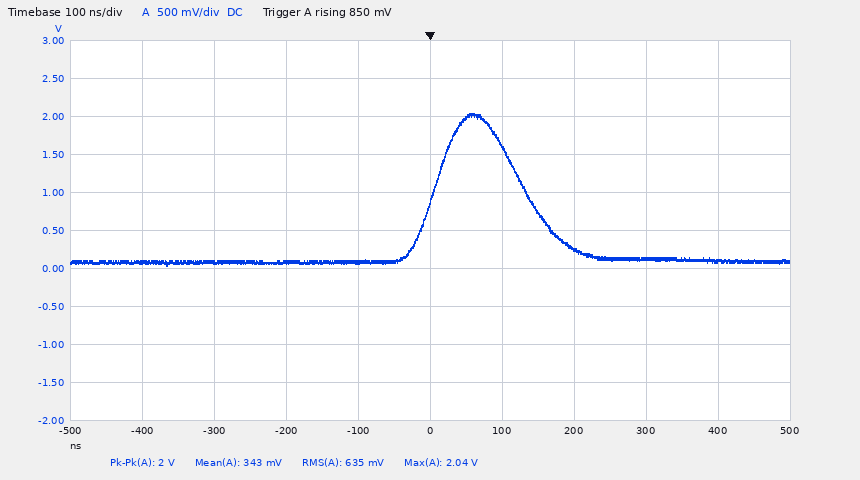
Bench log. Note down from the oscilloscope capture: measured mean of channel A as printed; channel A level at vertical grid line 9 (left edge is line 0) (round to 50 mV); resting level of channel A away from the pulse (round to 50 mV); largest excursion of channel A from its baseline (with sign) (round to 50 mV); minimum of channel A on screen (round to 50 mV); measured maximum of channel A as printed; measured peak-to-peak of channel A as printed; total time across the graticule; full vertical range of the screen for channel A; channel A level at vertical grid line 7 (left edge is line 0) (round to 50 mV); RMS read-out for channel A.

343 mV
100 mV
100 mV
+1.95 V
50 mV
2.04 V
2 V
1 µs
5 V
250 mV
635 mV
